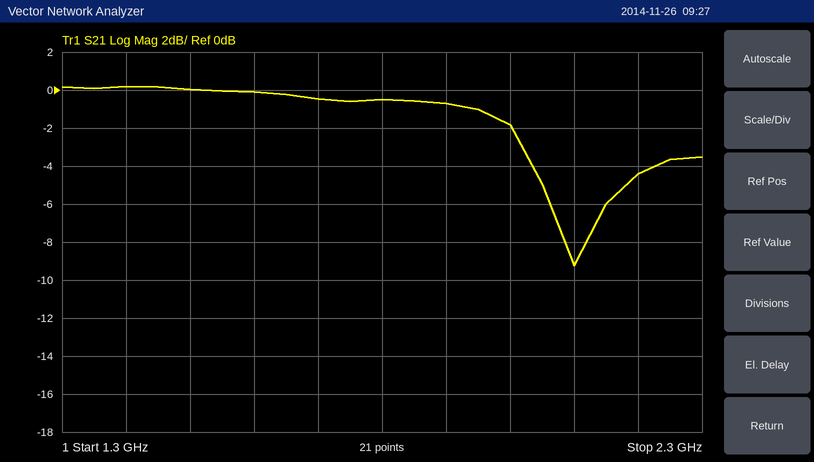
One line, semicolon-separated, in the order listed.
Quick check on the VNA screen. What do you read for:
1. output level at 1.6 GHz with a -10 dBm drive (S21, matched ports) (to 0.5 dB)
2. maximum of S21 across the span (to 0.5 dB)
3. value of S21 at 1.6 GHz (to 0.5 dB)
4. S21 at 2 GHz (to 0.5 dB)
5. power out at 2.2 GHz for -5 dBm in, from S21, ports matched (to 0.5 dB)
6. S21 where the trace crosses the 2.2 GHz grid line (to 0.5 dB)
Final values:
-10.0 dBm; 0.0 dB; 0.0 dB; -2.0 dB; -9.5 dBm; -4.5 dB
